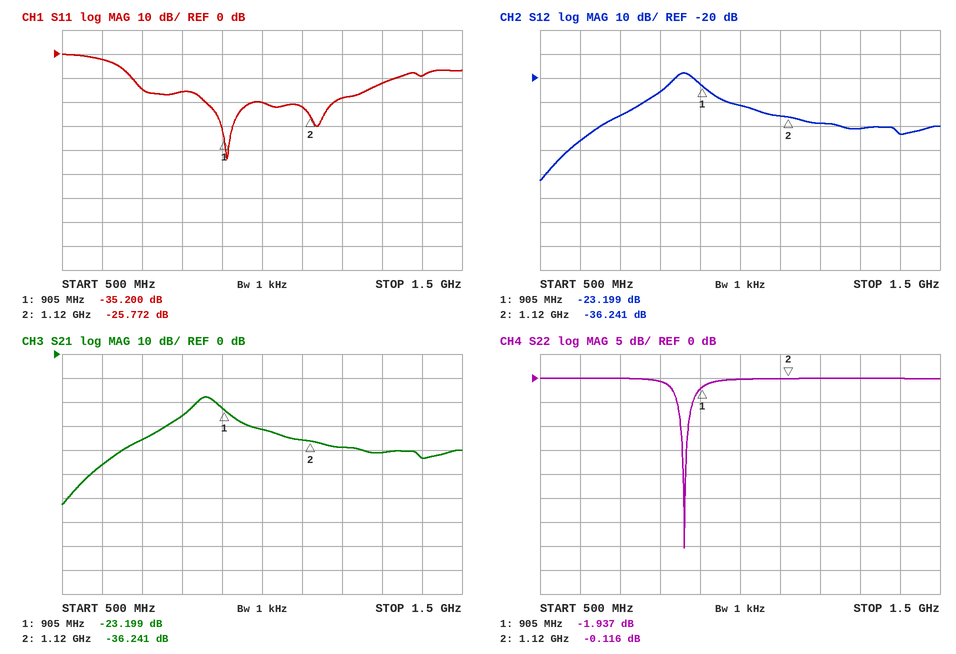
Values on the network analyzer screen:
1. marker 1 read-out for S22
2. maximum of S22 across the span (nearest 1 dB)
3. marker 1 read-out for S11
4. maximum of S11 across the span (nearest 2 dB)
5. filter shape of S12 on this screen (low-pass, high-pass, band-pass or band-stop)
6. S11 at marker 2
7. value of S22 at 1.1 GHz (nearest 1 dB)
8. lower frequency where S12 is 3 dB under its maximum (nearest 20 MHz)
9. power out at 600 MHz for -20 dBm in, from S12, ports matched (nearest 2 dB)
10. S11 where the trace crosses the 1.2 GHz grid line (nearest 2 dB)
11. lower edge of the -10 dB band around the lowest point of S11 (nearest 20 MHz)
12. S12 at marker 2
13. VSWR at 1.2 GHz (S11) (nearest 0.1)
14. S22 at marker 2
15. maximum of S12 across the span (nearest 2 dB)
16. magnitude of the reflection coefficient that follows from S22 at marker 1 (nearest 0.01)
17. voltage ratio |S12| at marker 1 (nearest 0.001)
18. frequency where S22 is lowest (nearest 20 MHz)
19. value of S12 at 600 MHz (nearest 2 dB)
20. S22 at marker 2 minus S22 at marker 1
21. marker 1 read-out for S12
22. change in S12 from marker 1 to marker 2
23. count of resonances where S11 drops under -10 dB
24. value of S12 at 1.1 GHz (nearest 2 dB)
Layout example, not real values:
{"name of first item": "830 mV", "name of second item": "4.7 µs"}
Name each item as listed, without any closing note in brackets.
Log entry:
{"marker 1 read-out for S22": "-1.937 dB", "maximum of S22 across the span": "0 dB", "marker 1 read-out for S11": "-35.200 dB", "maximum of S11 across the span": "0 dB", "filter shape of S12 on this screen": "band-pass", "S11 at marker 2": "-25.772 dB", "value of S22 at 1.1 GHz": "0 dB", "lower frequency where S12 is 3 dB under its maximum": "840 MHz", "power out at 600 MHz for -20 dBm in, from S12, ports matched": "-66 dBm", "S11 where the trace crosses the 1.2 GHz grid line": "-18 dB", "lower edge of the -10 dB band around the lowest point of S11": "680 MHz", "S12 at marker 2": "-36.241 dB", "VSWR at 1.2 GHz (S11)": "1.3", "S22 at marker 2": "-0.116 dB", "maximum of S12 across the span": "-18 dB", "magnitude of the reflection coefficient that follows from S22 at marker 1": "0.80", "voltage ratio |S12| at marker 1": "0.069", "frequency where S22 is lowest": "860 MHz", "value of S12 at 600 MHz": "-46 dB", "S22 at marker 2 minus S22 at marker 1": "1.821 dB", "marker 1 read-out for S12": "-23.199 dB", "change in S12 from marker 1 to marker 2": "-13.042 dB", "count of resonances where S11 drops under -10 dB": "2", "value of S12 at 1.1 GHz": "-36 dB"}
